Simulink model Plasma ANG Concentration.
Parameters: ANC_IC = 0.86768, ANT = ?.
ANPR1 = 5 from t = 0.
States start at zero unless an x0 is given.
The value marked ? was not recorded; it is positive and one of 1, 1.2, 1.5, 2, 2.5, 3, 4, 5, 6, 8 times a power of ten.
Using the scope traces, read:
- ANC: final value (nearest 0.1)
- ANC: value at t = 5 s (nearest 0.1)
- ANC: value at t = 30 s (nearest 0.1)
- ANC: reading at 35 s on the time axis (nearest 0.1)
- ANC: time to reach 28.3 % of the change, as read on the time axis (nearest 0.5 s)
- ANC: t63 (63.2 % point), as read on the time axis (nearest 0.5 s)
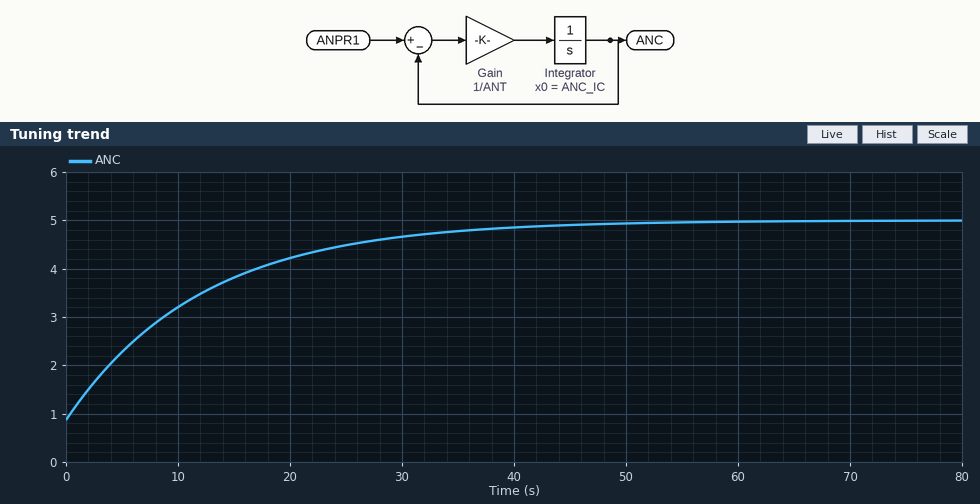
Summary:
5.0
2.3
4.7
4.8
4.0 s
12.0 s
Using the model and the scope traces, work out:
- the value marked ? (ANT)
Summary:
12
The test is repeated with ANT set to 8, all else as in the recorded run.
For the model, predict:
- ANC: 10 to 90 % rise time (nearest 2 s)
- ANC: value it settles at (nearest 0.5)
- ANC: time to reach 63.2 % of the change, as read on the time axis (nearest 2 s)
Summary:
18 s
5.0
8 s
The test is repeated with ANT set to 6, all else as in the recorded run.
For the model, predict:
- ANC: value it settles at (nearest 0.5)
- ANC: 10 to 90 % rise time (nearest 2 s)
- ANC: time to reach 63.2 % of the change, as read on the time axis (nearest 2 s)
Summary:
5.0
14 s
6 s
